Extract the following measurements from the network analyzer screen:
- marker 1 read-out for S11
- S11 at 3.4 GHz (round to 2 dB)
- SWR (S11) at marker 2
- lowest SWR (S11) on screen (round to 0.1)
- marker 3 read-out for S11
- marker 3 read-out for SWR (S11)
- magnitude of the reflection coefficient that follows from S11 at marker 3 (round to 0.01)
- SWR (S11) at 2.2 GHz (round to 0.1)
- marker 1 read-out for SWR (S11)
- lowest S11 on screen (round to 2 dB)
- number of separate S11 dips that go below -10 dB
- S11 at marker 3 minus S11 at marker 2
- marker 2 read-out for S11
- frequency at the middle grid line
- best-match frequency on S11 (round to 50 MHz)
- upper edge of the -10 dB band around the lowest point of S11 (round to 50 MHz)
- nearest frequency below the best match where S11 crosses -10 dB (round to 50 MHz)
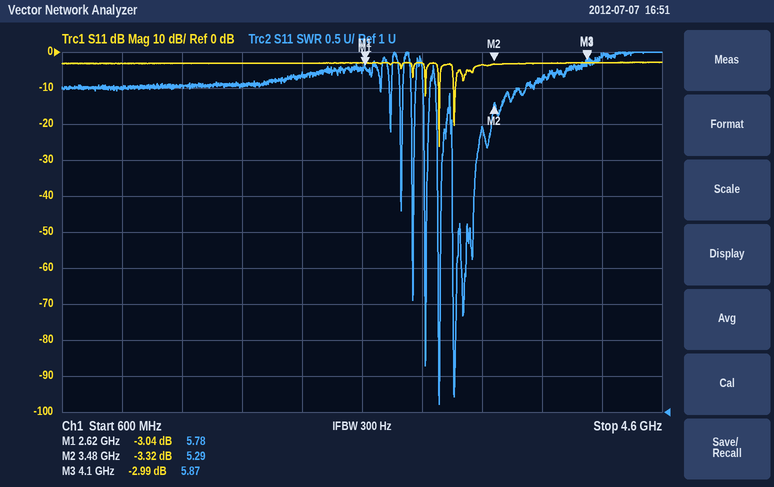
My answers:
-3.04 dB
-4 dB
5.29
1.1
-2.99 dB
5.87
0.71
5.7
5.78
-26 dB
3
0.33 dB
-3.32 dB
2.6 GHz
3.10 GHz
3.10 GHz
3.10 GHz
